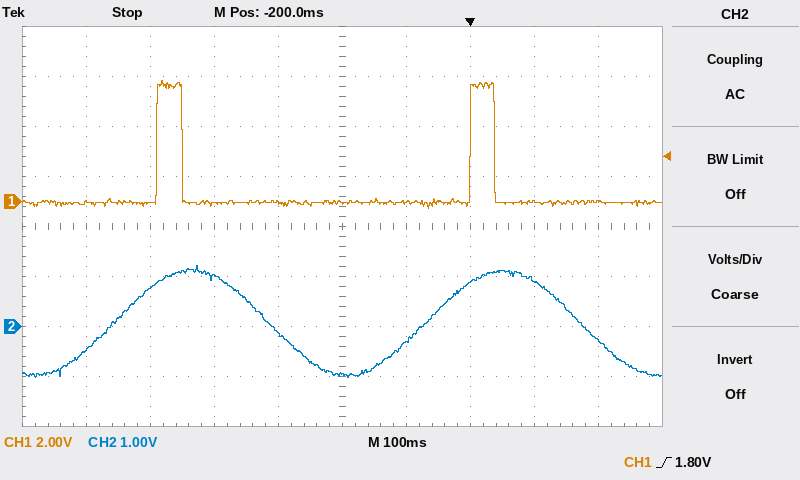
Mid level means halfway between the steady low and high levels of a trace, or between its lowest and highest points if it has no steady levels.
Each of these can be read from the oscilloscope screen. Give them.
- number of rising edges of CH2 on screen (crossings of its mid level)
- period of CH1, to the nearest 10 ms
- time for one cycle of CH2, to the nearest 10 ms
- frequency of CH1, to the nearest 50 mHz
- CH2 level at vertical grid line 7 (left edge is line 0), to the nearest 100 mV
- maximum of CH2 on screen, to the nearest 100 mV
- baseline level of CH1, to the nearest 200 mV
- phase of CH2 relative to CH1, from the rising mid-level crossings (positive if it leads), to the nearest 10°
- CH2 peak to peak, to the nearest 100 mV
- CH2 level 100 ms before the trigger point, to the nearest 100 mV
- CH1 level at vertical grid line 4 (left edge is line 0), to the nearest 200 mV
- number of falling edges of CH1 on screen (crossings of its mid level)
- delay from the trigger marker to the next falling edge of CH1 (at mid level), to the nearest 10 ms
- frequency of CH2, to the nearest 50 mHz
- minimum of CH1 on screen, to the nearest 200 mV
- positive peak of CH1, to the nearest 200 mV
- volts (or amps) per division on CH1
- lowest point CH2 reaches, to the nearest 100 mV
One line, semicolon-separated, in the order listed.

2; 490 ms; 490 ms; 2.05 Hz; 900 mV; 1.2 V; 0.0 V; +50°; 2.2 V; -300 mV; 0.0 V; 2; 40 ms; 2.05 Hz; -200 mV; 4.8 V; 2 V; -1.0 V
